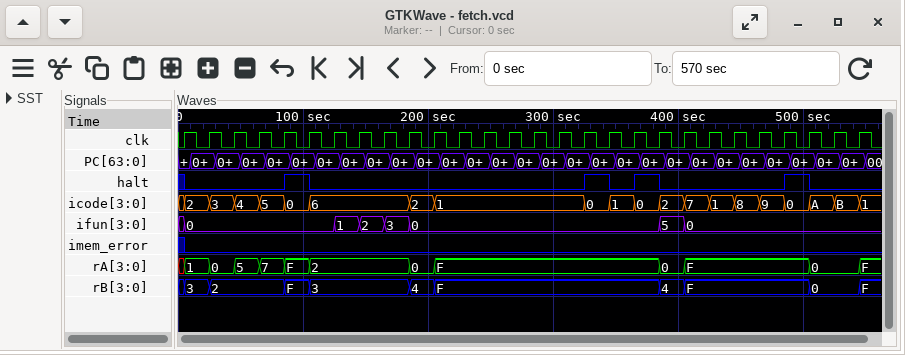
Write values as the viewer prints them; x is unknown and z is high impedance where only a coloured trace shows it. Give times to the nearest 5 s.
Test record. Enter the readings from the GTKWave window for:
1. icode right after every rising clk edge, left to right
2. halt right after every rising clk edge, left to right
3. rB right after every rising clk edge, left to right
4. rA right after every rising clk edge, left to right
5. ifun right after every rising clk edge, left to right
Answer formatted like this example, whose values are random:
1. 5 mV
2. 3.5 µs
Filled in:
1. 2, 3, 4, 5, 0, 6, 6, 6, 6, 2, 1, 1, 1, 1, 1, 1, 0, 1, 0, 2, 7, 1, 8, 9, 0, A, B, 1
2. 0 0 0 0 1 0 0 0 0 0 0 0 0 0 0 0 1 0 1 0 0 0 0 0 1 0 0 0
3. 3, 2, 2, 2, F, 3, 3, 3, 3, 4, F, F, F, F, F, F, F, F, F, 4, F, F, F, F, F, 0, 0, F
4. 1, 0, 5, 7, F, 2, 2, 2, 2, 0, F, F, F, F, F, F, F, F, F, 0, F, F, F, F, F, 0, 0, F
5. 0, 0, 0, 0, 0, 0, 1, 2, 3, 0, 0, 0, 0, 0, 0, 0, 0, 0, 0, 5, 0, 0, 0, 0, 0, 0, 0, 0
